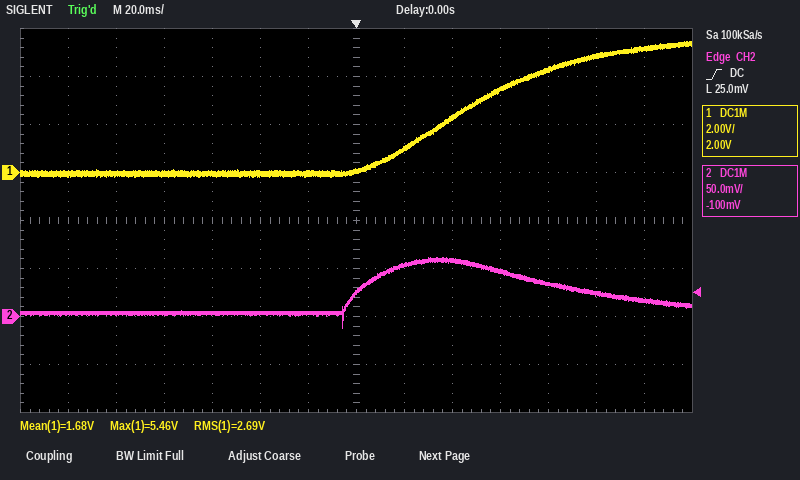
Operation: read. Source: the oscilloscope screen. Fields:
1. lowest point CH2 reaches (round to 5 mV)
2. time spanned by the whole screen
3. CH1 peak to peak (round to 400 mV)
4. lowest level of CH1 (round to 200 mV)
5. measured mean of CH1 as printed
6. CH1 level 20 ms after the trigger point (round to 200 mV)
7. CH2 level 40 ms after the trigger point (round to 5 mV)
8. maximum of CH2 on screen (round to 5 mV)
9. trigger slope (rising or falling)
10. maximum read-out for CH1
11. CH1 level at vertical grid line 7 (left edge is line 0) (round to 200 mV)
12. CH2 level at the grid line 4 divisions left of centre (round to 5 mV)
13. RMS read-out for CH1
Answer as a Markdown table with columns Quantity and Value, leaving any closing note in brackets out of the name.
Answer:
| Quantity | Value |
|---|---|
| lowest point CH2 reaches | -10 mV |
| time spanned by the whole screen | 280 ms |
| CH1 peak to peak | 5.6 V |
| lowest level of CH1 | -200 mV |
| measured mean of CH1 as printed | 1.68 V |
| CH1 level 20 ms after the trigger point | 1.0 V |
| CH2 level 40 ms after the trigger point | 60 mV |
| maximum of CH2 on screen | 60 mV |
| trigger slope | rising |
| maximum read-out for CH1 | 5.46 V |
| CH1 level at vertical grid line 7 (left edge is line 0) | 0.0 V |
| CH2 level at the grid line 4 divisions left of centre | 5 mV |
| RMS read-out for CH1 | 2.69 V |
